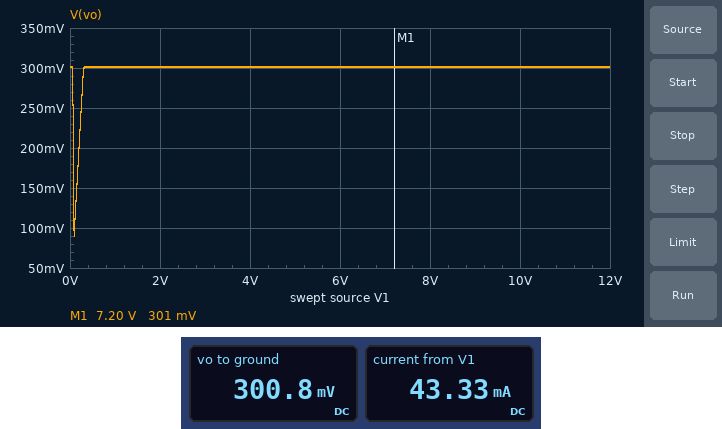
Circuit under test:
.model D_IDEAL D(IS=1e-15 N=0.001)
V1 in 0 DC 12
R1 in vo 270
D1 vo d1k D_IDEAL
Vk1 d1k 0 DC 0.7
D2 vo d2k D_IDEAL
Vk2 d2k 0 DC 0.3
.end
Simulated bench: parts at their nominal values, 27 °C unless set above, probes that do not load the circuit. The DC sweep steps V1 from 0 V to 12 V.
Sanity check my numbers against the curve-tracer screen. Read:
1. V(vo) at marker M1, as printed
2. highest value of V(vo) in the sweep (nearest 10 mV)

301 mV
300 mV
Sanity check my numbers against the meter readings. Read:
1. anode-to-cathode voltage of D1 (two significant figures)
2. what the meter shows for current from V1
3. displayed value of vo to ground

-400 mV
43.33 mA
300.8 mV
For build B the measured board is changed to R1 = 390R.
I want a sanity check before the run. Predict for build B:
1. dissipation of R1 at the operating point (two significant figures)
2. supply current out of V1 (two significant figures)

350 mW
30 mA
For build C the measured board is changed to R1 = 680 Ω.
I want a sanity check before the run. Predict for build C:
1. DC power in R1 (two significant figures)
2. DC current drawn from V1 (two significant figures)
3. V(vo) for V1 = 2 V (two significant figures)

200 mW
17 mA
300 mV
